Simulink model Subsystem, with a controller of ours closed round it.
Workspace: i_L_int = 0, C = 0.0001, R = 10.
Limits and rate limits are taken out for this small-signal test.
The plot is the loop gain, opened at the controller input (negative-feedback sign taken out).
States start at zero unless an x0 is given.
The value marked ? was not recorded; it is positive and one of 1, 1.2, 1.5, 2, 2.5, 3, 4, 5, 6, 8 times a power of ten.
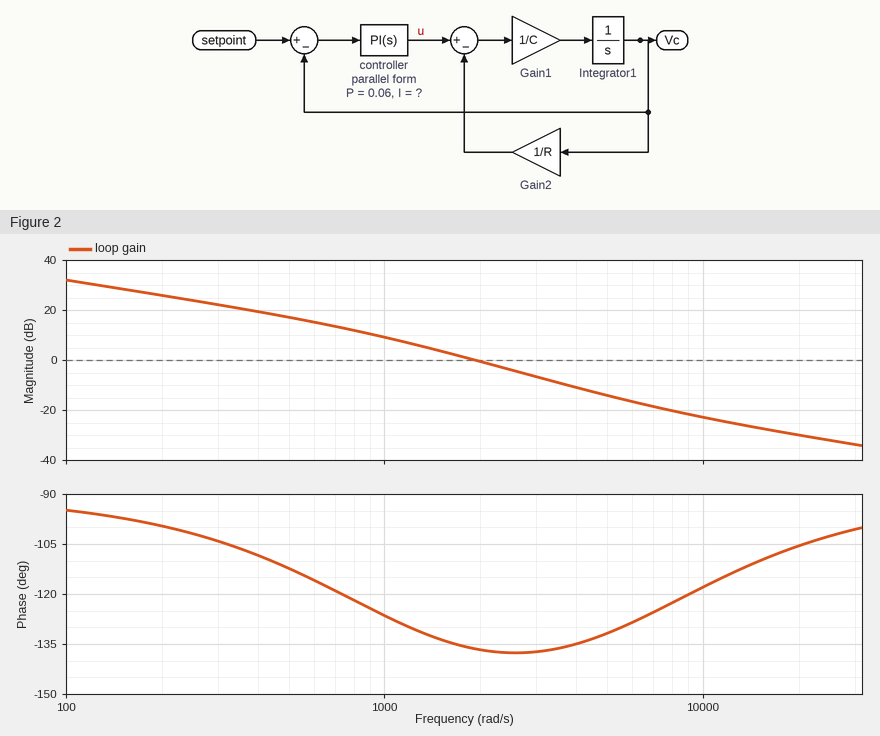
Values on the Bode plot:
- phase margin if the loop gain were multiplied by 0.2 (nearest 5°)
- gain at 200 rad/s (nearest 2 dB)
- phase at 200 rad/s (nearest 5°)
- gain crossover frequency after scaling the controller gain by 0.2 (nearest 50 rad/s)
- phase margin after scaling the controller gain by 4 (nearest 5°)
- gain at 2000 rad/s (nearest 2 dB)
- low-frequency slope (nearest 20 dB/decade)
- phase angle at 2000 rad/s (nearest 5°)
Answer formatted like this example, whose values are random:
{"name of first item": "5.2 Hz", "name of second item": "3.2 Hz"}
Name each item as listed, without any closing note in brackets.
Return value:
{"phase margin if the loop gain were multiplied by 0.2": "60°", "gain at 200 rad/s": "26 dB", "phase at 200 rad/s": "-100°", "gain crossover frequency after scaling the controller gain by 0.2": "650 rad/s", "phase margin after scaling the controller gain by 4": "45°", "gain at 2000 rad/s": "0 dB", "low-frequency slope": "-20 dB/decade", "phase angle at 2000 rad/s": "-135°"}
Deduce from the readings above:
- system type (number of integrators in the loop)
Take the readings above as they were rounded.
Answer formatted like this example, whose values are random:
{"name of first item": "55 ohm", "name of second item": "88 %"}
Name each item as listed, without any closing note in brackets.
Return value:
{"system type": "1"}
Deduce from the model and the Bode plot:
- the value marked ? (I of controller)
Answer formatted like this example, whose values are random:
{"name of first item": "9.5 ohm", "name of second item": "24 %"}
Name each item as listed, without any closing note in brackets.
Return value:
{"the value marked ?": "400"}
